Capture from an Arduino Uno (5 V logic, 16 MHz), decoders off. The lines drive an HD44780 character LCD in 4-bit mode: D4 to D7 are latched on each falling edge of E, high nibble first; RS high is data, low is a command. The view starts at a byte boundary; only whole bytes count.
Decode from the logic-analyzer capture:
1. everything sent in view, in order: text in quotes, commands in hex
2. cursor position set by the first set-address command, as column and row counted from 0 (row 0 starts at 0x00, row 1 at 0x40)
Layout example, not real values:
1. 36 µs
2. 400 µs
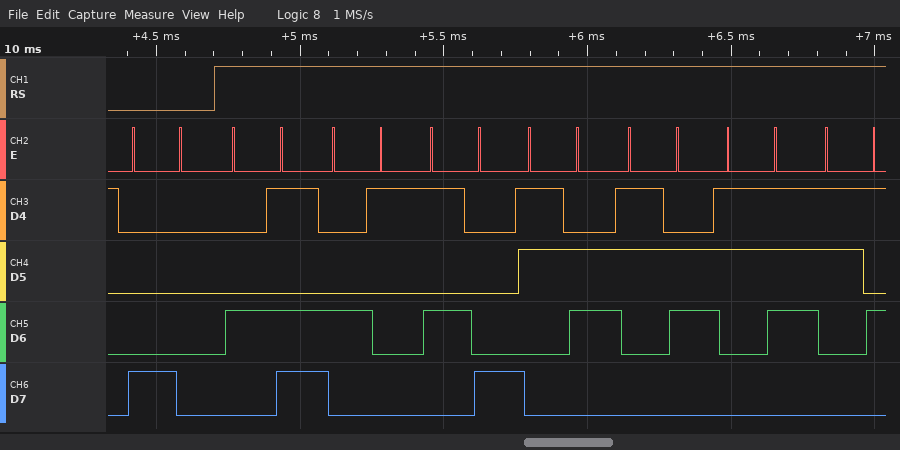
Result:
1. 0x80 "MAX6675"
2. column 0, row 0
